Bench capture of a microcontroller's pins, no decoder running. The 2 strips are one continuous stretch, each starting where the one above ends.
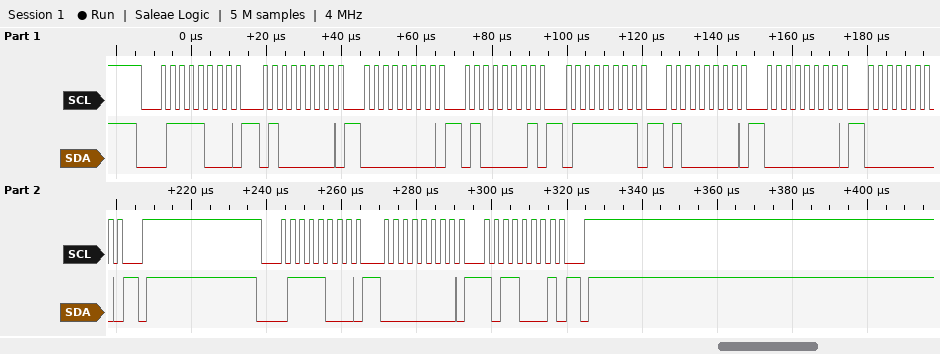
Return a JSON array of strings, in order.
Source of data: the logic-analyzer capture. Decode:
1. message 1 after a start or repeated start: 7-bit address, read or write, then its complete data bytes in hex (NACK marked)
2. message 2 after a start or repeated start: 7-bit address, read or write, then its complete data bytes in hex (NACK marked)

["0x3C write: 40 00 41 7F 40 00 00", "0x3C write: 00 B1"]
